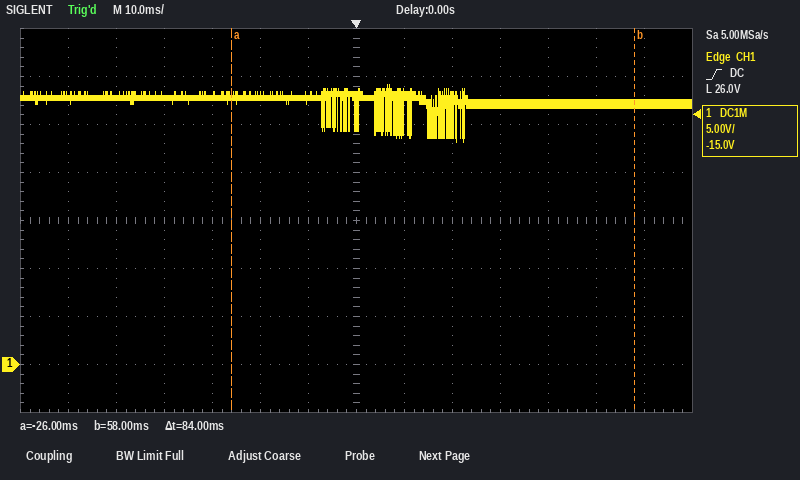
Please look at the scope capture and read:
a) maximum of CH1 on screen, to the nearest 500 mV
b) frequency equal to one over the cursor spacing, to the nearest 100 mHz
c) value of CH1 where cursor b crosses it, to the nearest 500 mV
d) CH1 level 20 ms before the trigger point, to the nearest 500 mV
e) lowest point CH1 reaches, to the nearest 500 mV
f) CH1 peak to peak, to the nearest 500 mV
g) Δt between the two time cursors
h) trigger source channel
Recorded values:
29.0 V
11.9 Hz
27.0 V
28.0 V
23.0 V
6.0 V
84 ms
CH1
